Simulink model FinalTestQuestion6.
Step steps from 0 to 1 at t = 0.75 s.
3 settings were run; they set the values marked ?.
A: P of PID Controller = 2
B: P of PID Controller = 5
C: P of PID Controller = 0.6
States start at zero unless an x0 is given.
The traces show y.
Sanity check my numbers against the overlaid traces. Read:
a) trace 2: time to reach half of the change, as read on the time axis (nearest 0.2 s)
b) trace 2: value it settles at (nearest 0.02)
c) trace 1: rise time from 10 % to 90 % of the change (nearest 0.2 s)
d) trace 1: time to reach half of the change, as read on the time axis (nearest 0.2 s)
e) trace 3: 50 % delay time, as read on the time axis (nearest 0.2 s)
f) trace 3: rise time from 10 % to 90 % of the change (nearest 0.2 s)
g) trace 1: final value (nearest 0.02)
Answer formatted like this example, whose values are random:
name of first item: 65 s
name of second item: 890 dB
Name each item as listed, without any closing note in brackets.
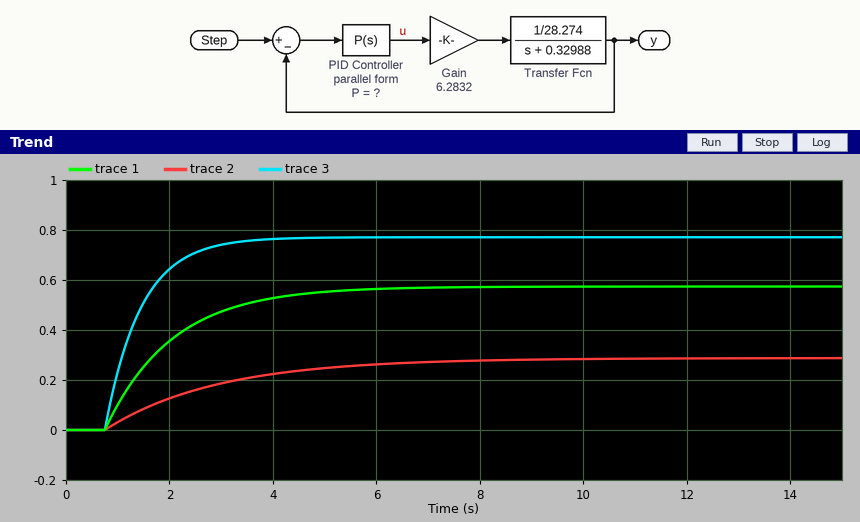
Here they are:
trace 2: time to reach half of the change, as read on the time axis: 2.2 s
trace 2: value it settles at: 0.28
trace 1: rise time from 10 % to 90 % of the change: 2.8 s
trace 1: time to reach half of the change, as read on the time axis: 1.6 s
trace 3: 50 % delay time, as read on the time axis: 1.2 s
trace 3: rise time from 10 % to 90 % of the change: 1.6 s
trace 1: final value: 0.58
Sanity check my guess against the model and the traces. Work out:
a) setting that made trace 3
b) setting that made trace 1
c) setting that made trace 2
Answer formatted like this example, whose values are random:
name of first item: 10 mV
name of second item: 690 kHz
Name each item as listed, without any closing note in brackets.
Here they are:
setting that made trace 3: B
setting that made trace 1: A
setting that made trace 2: C
